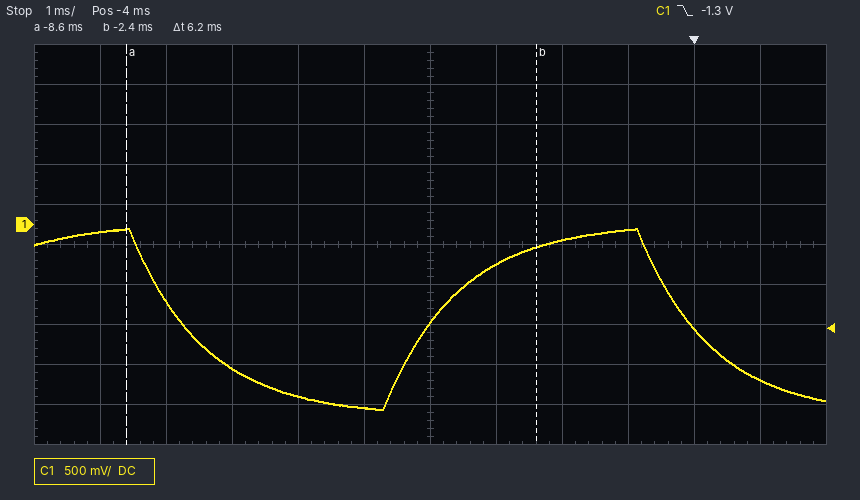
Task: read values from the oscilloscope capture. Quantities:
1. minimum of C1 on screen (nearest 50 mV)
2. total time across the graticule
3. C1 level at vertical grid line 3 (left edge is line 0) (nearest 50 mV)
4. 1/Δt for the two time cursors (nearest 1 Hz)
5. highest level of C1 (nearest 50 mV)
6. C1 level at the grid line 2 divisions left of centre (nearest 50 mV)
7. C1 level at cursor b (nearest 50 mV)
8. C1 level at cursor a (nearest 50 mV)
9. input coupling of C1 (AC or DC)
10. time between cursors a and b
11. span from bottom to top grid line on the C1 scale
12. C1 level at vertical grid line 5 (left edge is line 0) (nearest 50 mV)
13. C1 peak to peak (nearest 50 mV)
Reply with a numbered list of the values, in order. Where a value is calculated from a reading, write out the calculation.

1. -2.30 V
2. 12 ms
3. -1.80 V
4. 1 / 6.2 ms ≈ 161 Hz
5. -50 mV
6. -2.15 V
7. -300 mV
8. -50 mV
9. DC
10. 6.2 ms
11. 5 V
12. -2.30 V
13. -50 mV − (-2.30 V) = 2.25 V
